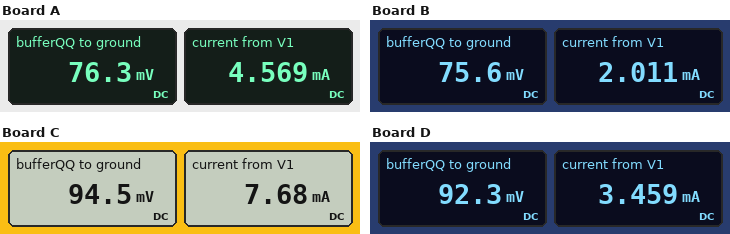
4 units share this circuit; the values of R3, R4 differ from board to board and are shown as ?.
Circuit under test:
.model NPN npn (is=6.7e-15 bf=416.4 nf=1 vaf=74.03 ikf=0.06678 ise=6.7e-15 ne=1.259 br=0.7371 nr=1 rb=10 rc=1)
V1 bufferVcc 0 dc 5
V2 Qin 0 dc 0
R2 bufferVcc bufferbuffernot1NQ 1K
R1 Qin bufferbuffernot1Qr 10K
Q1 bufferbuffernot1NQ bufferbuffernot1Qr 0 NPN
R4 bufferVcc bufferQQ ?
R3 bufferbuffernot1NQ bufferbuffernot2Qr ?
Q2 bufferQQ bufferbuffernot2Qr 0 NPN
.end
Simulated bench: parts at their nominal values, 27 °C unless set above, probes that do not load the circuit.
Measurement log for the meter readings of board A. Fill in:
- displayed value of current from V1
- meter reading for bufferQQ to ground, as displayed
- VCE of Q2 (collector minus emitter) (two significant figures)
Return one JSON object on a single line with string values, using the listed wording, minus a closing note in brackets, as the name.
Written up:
{"displayed value of current from V1": "4.569 mA", "meter reading for bufferQQ to ground, as displayed": "76.3 mV", "VCE of Q2 (collector minus emitter)": "76 mV"}
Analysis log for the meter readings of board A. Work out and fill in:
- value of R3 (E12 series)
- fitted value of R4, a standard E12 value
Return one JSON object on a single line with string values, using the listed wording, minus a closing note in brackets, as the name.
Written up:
{"value of R3": "8.2 kΩ", "fitted value of R4, a standard E12 value": "1.2 kΩ"}
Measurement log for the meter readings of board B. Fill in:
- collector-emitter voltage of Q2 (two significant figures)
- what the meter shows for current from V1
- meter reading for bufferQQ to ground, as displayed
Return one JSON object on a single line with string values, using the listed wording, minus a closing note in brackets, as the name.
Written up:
{"collector-emitter voltage of Q2": "76 mV", "what the meter shows for current from V1": "2.011 mA", "meter reading for bufferQQ to ground, as displayed": "75.6 mV"}
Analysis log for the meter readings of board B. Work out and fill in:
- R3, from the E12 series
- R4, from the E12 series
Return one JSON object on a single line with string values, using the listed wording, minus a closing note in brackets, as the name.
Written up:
{"R3, from the E12 series": "22 kΩ", "R4, from the E12 series": "2.7 kΩ"}
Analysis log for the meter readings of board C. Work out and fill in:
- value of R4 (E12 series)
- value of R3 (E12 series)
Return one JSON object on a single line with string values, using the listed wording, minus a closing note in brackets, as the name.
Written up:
{"value of R4": "680 Ω", "value of R3": "8.2 kΩ"}
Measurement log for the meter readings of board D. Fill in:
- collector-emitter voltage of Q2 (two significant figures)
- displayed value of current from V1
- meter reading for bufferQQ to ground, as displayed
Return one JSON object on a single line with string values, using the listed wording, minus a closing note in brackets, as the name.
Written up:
{"collector-emitter voltage of Q2": "92 mV", "displayed value of current from V1": "3.459 mA", "meter reading for bufferQQ to ground, as displayed": "92.3 mV"}
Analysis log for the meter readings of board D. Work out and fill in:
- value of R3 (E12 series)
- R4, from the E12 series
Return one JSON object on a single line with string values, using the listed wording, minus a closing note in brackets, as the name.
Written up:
{"value of R3": "22 kΩ", "R4, from the E12 series": "1.5 kΩ"}
